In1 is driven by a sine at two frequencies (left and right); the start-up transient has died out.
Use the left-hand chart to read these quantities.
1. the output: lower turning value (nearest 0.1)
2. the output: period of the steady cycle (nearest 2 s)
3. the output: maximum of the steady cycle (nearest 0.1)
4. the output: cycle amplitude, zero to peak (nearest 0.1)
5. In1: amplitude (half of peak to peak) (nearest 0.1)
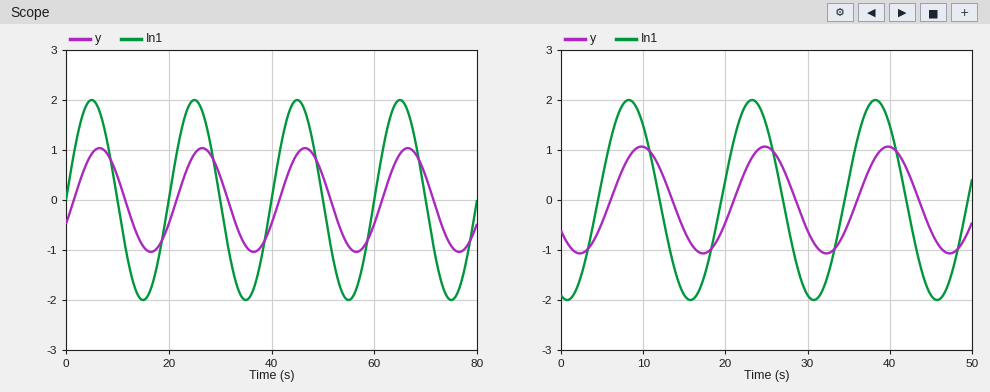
-1.0
20 s
1.0
1.0
2.0
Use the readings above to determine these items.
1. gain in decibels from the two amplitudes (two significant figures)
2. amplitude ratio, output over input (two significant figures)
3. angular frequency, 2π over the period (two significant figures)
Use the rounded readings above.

-6.0 dB
0.50
0.31 rad/s
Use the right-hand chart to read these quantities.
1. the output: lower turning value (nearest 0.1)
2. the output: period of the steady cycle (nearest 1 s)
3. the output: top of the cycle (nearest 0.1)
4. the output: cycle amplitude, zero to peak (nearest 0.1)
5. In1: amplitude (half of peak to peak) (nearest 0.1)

-1.1
15 s
1.1
1.1
2.0
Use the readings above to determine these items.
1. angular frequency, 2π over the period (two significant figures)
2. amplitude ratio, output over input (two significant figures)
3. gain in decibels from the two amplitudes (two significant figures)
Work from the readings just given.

0.42 rad/s
0.55
-5.2 dB
